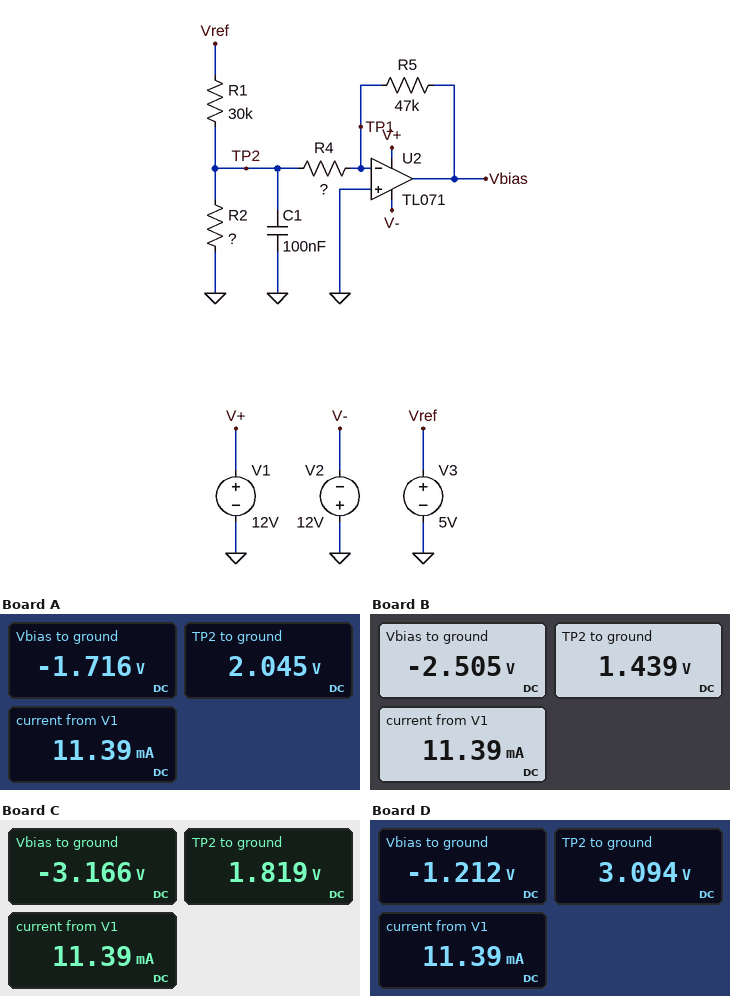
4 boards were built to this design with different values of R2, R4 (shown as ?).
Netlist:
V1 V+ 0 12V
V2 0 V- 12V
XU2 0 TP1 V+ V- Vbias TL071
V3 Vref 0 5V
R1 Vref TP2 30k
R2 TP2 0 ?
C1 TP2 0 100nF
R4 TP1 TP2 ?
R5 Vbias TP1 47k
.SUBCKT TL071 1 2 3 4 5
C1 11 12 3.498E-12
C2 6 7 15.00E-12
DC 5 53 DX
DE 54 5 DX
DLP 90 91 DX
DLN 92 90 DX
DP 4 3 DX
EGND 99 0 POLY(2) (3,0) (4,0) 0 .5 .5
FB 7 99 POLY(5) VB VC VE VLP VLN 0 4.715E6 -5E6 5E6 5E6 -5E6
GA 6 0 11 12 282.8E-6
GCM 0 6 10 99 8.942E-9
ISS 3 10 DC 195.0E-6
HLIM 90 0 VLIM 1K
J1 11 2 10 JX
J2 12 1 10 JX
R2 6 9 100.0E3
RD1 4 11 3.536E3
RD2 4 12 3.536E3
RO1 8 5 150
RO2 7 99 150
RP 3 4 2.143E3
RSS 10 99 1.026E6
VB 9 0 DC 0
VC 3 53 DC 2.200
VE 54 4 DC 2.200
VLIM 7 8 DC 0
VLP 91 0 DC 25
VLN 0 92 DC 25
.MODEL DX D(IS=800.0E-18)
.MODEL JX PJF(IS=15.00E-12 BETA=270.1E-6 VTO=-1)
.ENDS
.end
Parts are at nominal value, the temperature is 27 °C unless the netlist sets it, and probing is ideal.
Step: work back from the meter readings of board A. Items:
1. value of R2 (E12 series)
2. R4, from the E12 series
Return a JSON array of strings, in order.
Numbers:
["33 kΩ", "56 kΩ"]
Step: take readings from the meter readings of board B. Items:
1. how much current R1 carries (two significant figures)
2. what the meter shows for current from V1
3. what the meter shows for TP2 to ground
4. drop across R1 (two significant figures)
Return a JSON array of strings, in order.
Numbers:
["120 µA", "11.39 mA", "1.439 V", "3.6 V"]
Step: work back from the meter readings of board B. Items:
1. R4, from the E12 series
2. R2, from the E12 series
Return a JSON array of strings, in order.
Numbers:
["27 kΩ", "22 kΩ"]
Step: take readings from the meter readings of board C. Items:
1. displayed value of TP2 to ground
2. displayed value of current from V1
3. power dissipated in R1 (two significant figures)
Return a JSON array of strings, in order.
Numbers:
["1.819 V", "11.39 mA", "340 µW"]
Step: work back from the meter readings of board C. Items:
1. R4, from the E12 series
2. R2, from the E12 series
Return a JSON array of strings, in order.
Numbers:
["27 kΩ", "47 kΩ"]
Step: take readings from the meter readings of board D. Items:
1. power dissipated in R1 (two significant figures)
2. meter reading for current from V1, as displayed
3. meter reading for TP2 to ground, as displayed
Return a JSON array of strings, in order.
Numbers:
["120 µW", "11.39 mA", "3.094 V"]
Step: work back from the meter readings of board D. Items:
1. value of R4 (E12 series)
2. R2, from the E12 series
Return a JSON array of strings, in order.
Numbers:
["120 kΩ", "82 kΩ"]
